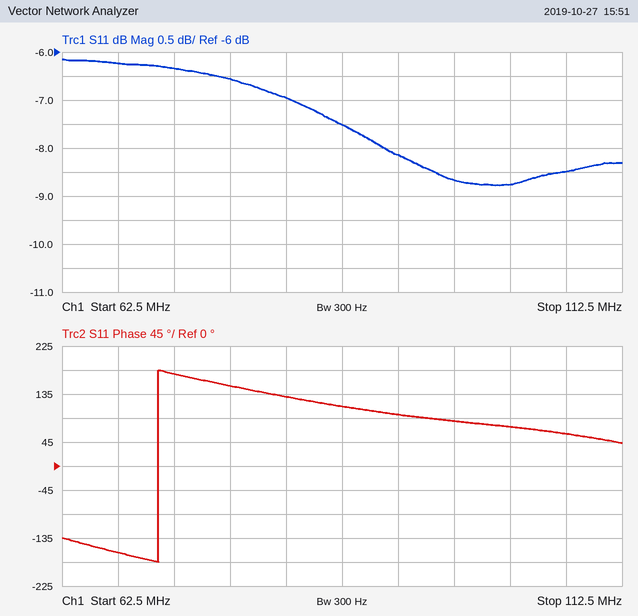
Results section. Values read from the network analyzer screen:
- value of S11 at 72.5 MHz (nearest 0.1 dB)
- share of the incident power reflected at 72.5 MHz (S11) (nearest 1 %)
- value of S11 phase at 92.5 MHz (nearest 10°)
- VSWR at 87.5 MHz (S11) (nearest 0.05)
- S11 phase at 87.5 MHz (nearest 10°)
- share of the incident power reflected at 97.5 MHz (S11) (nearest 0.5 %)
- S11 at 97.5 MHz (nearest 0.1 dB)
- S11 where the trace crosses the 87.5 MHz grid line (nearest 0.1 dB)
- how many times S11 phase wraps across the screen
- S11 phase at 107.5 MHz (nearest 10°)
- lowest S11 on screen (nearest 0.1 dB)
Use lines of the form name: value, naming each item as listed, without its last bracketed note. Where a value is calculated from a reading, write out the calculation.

value of S11 at 72.5 MHz: -6.3 dB
share of the incident power reflected at 72.5 MHz (S11): 10^(-6.3/10) ≈ 23 %
value of S11 phase at 92.5 MHz: 100°
VSWR at 87.5 MHz (S11): |Γ| = 10^(-7.5/20) = 0.4217; VSWR = (1 + 0.4217)/(1 − 0.4217) ≈ 2.46, so 2.45 to the nearest 0.05
S11 phase at 87.5 MHz: 110°
share of the incident power reflected at 97.5 MHz (S11): 10^(-8.7/10) ≈ 13.5 %
S11 at 97.5 MHz: -8.7 dB
S11 where the trace crosses the 87.5 MHz grid line: -7.5 dB
how many times S11 phase wraps across the screen: 1
S11 phase at 107.5 MHz: 60°
lowest S11 on screen: -8.8 dB
